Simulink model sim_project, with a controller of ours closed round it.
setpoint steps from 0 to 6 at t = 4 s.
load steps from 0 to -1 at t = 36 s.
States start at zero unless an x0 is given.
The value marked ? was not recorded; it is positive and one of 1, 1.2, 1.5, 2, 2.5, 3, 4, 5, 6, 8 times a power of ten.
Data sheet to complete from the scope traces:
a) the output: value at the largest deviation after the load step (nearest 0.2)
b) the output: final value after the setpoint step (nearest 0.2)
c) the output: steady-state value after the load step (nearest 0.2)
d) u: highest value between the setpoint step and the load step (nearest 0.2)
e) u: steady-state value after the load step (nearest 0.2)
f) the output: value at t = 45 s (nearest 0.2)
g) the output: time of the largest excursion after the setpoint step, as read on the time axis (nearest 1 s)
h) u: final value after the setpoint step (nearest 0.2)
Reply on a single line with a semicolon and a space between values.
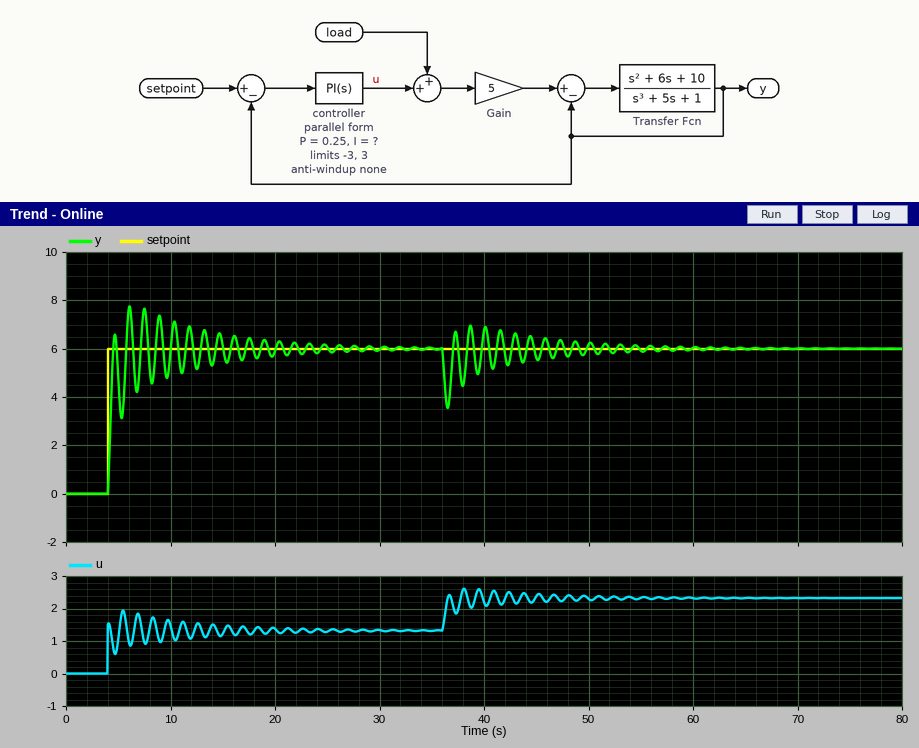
3.6; 6.0; 6.0; 2.0; 2.4; 5.6; 6 s; 1.4
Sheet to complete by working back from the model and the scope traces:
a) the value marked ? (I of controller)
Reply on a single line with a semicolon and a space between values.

0.5
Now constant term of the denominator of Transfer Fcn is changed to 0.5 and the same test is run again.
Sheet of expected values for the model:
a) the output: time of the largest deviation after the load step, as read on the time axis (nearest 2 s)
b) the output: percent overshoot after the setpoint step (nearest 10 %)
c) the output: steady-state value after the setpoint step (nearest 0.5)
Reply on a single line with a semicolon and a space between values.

36 s; 30 %; 6.0
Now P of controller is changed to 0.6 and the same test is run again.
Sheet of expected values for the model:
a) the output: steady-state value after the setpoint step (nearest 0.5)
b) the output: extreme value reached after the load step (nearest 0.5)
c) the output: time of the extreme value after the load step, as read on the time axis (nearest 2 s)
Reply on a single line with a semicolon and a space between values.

6.0; 4.5; 36 s
